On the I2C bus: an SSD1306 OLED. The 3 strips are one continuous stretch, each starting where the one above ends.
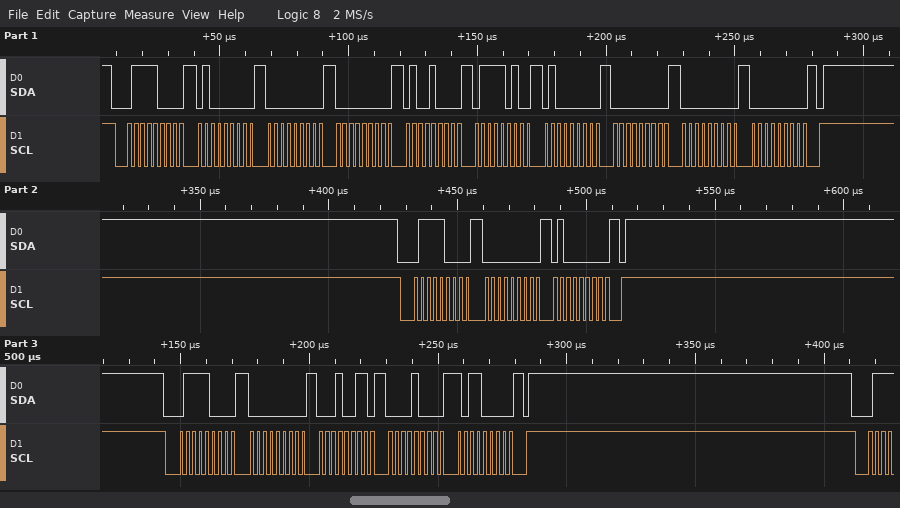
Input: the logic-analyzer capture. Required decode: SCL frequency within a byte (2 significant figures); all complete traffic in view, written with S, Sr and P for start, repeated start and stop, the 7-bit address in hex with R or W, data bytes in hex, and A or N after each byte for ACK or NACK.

400 kHz
S 3CW A 40 A 00 A 00 A 48 A 7A A 40 A 00 A 00 A 00 A P S 3CW A 00 A 40 A P S 3CW A 00 A 13 A 08 A B0 A P
